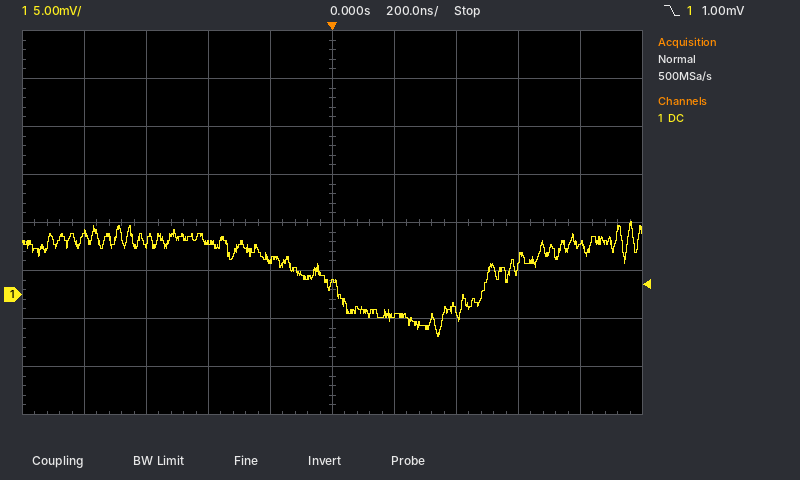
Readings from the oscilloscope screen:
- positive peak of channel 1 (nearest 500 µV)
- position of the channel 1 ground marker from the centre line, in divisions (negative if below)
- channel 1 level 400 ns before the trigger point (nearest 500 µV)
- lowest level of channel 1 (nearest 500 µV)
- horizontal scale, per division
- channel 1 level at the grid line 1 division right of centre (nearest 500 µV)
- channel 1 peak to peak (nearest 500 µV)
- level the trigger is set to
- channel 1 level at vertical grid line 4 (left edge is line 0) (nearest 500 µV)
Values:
7.5 mV
-1.5 div
5.5 mV
-4.5 mV
200 ns
-2.0 mV
12.0 mV
1.00 mV
3.5 mV
